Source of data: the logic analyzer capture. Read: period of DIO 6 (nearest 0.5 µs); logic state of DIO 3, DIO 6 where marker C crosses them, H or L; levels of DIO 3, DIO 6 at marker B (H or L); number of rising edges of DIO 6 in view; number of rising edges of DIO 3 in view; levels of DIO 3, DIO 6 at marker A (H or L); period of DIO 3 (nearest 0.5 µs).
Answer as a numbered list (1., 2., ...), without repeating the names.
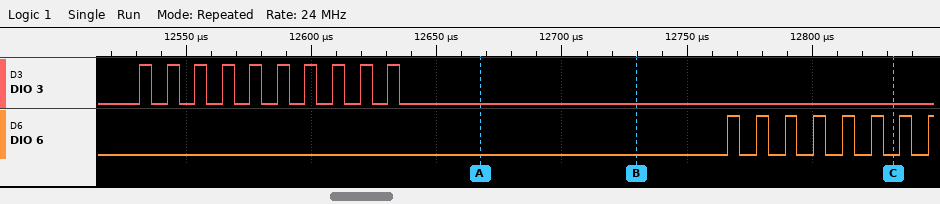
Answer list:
1. 11.5 µs
2. DIO 3=L, DIO 6=L
3. DIO 3=L, DIO 6=L
4. 8
5. 10
6. DIO 3=L, DIO 6=L
7. 11 µs
